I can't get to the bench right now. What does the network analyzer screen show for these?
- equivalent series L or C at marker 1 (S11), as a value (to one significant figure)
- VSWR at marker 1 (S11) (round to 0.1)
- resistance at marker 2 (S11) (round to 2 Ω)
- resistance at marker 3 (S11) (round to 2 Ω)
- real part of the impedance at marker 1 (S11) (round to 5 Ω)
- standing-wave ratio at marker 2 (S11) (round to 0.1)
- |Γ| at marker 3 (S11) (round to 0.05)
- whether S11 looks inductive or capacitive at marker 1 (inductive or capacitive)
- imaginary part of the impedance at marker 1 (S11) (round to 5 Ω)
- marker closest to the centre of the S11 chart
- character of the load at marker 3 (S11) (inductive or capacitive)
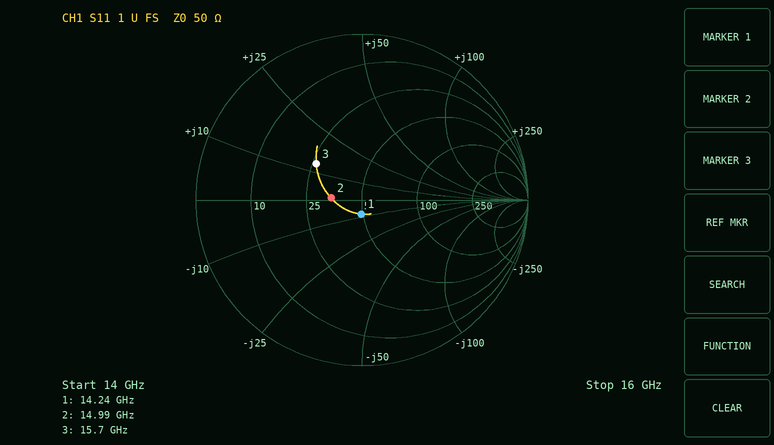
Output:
1 pF
1.2
34 Ω
26 Ω
50 Ω
1.5
0.35
capacitive
-10 Ω
marker 1
inductive
